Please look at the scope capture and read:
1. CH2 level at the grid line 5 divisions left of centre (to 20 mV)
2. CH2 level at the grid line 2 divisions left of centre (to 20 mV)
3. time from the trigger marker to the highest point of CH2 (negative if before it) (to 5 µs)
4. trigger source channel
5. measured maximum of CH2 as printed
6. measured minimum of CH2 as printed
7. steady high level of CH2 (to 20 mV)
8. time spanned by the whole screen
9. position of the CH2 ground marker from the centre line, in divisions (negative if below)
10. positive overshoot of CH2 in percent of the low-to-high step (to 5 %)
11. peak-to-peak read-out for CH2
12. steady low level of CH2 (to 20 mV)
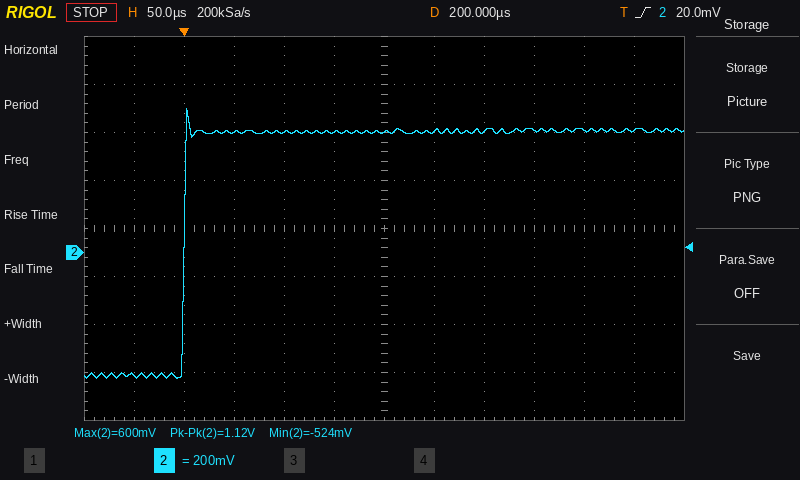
-520 mV
500 mV
+5 µs
CH2
600 mV
-524 mV
500 mV
600 µs
-0.5 div
10 %
1.12 V
-520 mV
